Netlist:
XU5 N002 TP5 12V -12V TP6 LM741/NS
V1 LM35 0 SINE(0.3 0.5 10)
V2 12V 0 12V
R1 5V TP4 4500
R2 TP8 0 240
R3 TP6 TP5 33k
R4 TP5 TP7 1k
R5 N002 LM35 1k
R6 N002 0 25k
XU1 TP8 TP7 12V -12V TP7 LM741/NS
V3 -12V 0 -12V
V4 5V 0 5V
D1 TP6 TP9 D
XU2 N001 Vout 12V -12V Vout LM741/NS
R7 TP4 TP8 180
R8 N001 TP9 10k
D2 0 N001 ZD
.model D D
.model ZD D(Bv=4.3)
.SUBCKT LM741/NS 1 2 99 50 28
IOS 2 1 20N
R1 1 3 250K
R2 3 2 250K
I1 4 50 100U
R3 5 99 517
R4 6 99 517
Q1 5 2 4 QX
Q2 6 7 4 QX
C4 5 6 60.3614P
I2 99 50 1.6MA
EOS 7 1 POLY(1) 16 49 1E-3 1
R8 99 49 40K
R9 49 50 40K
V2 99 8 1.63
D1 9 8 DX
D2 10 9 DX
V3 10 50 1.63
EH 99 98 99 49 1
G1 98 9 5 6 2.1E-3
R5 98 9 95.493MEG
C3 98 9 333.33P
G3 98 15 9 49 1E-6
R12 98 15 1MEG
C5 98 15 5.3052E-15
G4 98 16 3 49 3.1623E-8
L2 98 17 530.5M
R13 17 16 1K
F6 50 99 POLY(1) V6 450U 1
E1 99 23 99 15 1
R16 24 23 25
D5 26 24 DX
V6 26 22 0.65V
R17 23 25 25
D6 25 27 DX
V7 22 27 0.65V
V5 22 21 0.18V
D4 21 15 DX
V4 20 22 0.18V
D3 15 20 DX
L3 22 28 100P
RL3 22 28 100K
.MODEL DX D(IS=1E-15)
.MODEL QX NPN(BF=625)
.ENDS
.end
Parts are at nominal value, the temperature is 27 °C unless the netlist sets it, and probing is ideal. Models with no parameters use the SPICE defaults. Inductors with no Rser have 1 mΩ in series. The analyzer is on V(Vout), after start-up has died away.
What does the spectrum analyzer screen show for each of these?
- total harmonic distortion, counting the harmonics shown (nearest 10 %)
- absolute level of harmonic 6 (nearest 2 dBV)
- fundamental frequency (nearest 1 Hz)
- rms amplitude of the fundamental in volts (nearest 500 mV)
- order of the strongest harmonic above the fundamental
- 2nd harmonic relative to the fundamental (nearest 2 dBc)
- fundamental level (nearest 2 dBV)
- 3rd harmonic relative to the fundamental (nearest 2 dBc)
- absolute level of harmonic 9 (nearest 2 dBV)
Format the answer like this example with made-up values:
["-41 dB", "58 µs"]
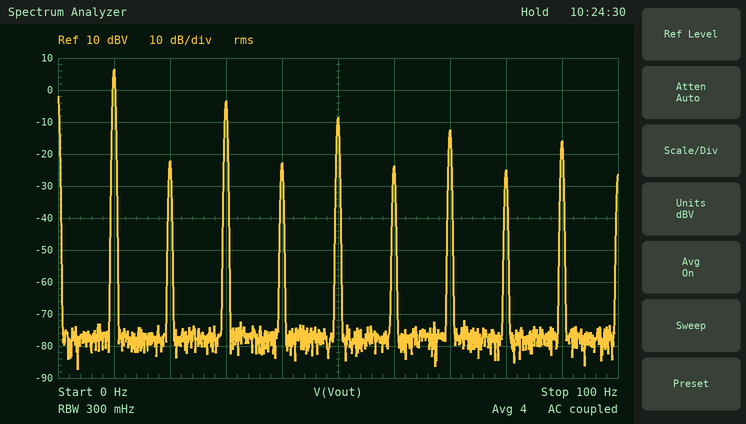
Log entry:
["40 %", "-24 dBV", "10 Hz", "2.0 V", "3", "-28 dBc", "6 dBV", "-10 dBc", "-16 dBV"]
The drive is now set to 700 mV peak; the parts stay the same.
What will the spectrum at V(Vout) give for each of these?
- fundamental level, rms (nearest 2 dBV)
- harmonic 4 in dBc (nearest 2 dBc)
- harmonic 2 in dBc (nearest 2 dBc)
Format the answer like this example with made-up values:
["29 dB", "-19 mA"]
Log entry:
["6 dBV", "-32 dBc", "-32 dBc"]
